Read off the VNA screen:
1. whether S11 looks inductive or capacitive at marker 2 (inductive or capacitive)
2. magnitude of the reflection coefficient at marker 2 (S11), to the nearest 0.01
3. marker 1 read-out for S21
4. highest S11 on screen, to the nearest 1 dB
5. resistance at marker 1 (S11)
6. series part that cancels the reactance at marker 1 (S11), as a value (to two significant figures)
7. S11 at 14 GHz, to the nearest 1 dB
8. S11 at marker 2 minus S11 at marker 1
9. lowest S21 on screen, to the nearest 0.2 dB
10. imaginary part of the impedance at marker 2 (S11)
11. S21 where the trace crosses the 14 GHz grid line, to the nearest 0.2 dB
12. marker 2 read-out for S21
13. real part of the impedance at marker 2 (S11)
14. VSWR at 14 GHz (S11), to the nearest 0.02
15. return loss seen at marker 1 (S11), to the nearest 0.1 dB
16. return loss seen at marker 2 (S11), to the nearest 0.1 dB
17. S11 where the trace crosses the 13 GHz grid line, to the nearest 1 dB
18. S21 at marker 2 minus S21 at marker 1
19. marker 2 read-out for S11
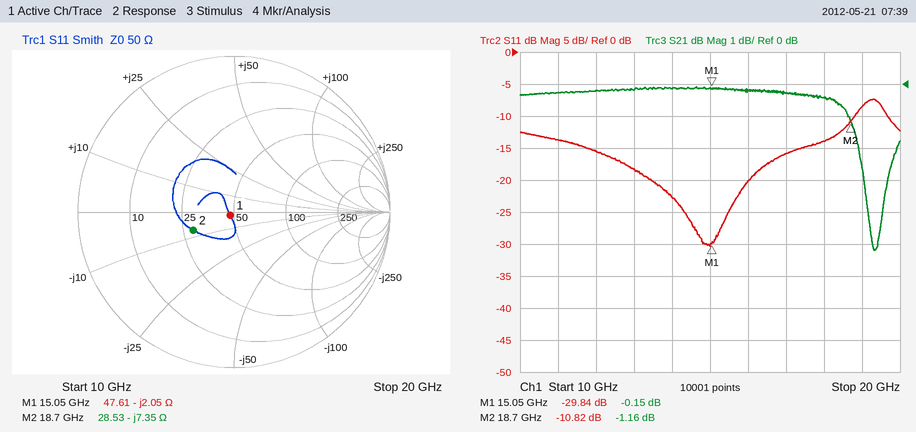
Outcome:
capacitive
0.29
-0.15 dB
-7 dB
47.61 Ω
22 pH
-23 dB
19.02 dB
-5.2 dB
-7.35 Ω
-0.2 dB
-1.16 dB
28.53 Ω
1.16
29.8 dB
10.8 dB
-18 dB
-1.01 dB
-10.82 dB
